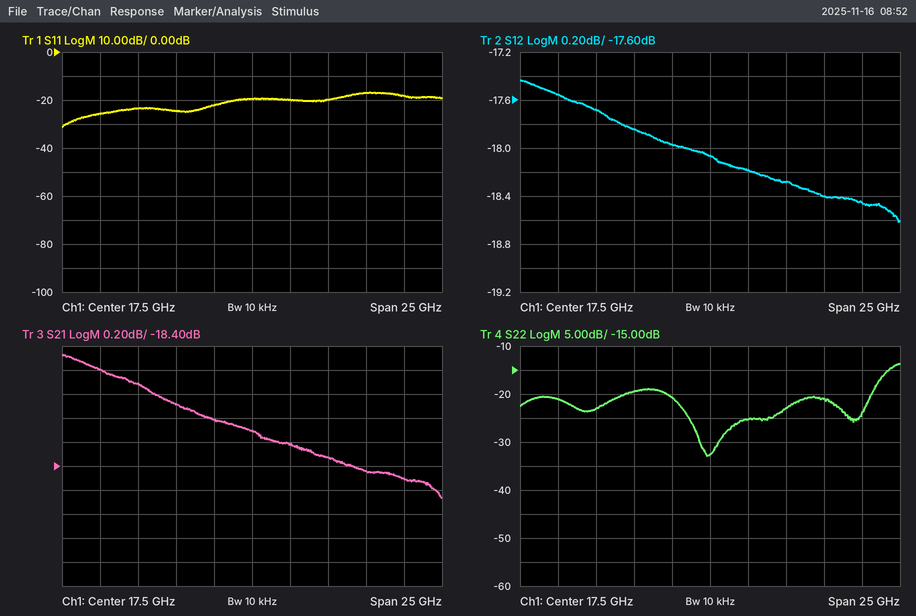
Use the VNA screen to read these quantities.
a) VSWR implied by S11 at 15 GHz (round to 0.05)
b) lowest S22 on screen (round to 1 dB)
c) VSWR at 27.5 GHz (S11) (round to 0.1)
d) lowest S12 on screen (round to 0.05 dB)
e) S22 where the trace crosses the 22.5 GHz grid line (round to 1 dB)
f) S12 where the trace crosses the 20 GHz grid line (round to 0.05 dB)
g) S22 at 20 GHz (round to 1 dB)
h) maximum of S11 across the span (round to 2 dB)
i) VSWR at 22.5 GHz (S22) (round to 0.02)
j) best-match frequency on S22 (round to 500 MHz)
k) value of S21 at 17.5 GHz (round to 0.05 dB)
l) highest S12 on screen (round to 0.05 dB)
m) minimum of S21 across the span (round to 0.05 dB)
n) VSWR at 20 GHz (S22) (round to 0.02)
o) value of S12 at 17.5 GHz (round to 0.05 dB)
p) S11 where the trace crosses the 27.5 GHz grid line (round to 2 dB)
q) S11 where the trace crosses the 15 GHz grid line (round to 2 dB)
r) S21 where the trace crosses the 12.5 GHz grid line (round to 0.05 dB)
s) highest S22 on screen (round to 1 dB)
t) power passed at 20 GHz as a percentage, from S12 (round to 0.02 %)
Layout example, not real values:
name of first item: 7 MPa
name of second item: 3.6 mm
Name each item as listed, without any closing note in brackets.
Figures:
VSWR implied by S11 at 15 GHz: 1.15
lowest S22 on screen: -33 dB
VSWR at 27.5 GHz (S11): 1.3
lowest S12 on screen: -18.60 dB
S22 where the trace crosses the 22.5 GHz grid line: -23 dB
S12 where the trace crosses the 20 GHz grid line: -18.20 dB
S22 at 20 GHz: -25 dB
maximum of S11 across the span: -16 dB
VSWR at 22.5 GHz (S22): 1.16
best-match frequency on S22: 17.5 GHz
value of S21 at 17.5 GHz: -18.10 dB
highest S12 on screen: -17.45 dB
minimum of S21 across the span: -18.65 dB
VSWR at 20 GHz (S22): 1.12
value of S12 at 17.5 GHz: -18.05 dB
S11 where the trace crosses the 27.5 GHz grid line: -18 dB
S11 where the trace crosses the 15 GHz grid line: -22 dB
S21 where the trace crosses the 12.5 GHz grid line: -17.90 dB
highest S22 on screen: -14 dB
power passed at 20 GHz as a percentage, from S12: 1.52 %
